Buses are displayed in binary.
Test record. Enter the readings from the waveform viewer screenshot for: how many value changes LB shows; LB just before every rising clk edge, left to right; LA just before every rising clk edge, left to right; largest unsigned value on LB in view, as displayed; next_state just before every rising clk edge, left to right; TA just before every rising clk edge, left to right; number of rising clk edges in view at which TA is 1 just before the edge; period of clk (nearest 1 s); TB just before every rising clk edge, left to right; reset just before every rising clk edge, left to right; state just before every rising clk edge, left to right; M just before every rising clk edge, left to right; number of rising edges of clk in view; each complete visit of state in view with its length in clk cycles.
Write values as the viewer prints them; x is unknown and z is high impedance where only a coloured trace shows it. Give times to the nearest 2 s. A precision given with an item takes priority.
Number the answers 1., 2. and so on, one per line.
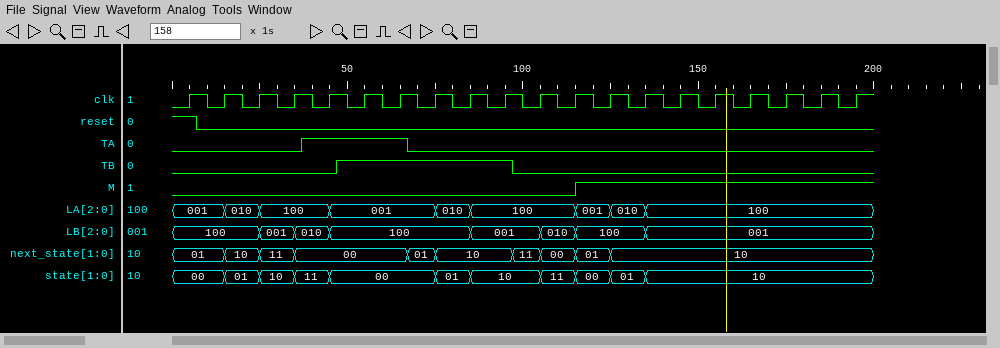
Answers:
1. 7
2. 100, 100, 100, 001, 010, 100, 100, 100, 100, 001, 001, 010, 100, 100, 001, 001, 001, 001, 001, 001
3. 001, 001, 010, 100, 100, 001, 001, 001, 010, 100, 100, 100, 001, 010, 100, 100, 100, 100, 100, 100
4. 100
5. 01, 01, 10, 11, 00, 00, 00, 01, 10, 10, 11, 00, 01, 10, 10, 10, 10, 10, 10, 10
6. 0 0 0 0 1 1 1 0 0 0 0 0 0 0 0 0 0 0 0 0
7. 3
8. 10 s
9. 0 0 0 0 0 1 1 1 1 1 0 0 0 0 0 0 0 0 0 0
10. 1 0 0 0 0 0 0 0 0 0 0 0 0 0 0 0 0 0 0 0
11. 00, 00, 01, 10, 11, 00, 00, 00, 01, 10, 10, 11, 00, 01, 10, 10, 10, 10, 10, 10
12. 0 0 0 0 0 0 0 0 0 0 0 0 1 1 1 1 1 1 1 1
13. 20
14. 01: 1, 10: 1, 11: 1, 00: 3, 01: 1, 10: 2, 11: 1, 00: 1, 01: 1
